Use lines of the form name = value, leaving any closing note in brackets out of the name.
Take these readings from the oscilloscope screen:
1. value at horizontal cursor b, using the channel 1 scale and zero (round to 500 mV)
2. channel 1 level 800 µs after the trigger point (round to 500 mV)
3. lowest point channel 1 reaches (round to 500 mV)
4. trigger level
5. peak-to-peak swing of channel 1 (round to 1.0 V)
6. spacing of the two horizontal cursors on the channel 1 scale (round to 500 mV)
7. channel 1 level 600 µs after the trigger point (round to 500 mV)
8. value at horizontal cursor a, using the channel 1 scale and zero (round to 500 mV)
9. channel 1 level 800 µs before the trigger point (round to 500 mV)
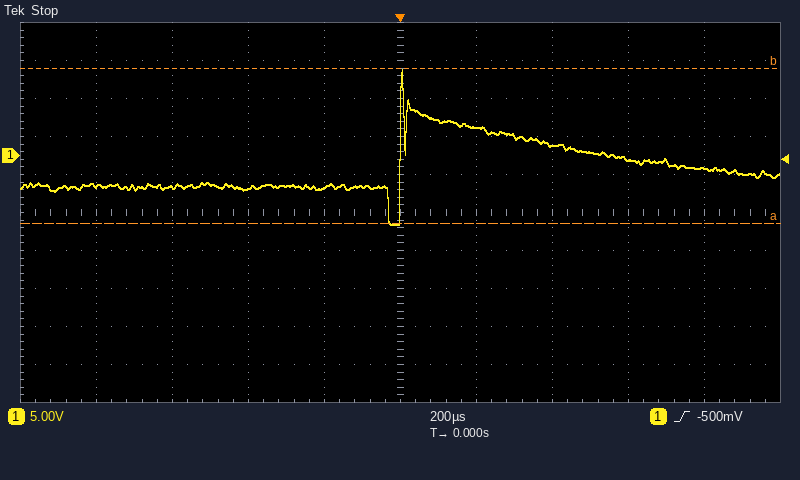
value at horizontal cursor b, using the channel 1 scale and zero = 11.5 V
channel 1 level 800 µs after the trigger point = -1.5 V
lowest point channel 1 reaches = -9.0 V
trigger level = -500 mV
peak-to-peak swing of channel 1 = 20.0 V
spacing of the two horizontal cursors on the channel 1 scale = 20.5 V
channel 1 level 600 µs after the trigger point = -500 mV
value at horizontal cursor a, using the channel 1 scale and zero = -9.0 V
channel 1 level 800 µs before the trigger point = -4.0 V
